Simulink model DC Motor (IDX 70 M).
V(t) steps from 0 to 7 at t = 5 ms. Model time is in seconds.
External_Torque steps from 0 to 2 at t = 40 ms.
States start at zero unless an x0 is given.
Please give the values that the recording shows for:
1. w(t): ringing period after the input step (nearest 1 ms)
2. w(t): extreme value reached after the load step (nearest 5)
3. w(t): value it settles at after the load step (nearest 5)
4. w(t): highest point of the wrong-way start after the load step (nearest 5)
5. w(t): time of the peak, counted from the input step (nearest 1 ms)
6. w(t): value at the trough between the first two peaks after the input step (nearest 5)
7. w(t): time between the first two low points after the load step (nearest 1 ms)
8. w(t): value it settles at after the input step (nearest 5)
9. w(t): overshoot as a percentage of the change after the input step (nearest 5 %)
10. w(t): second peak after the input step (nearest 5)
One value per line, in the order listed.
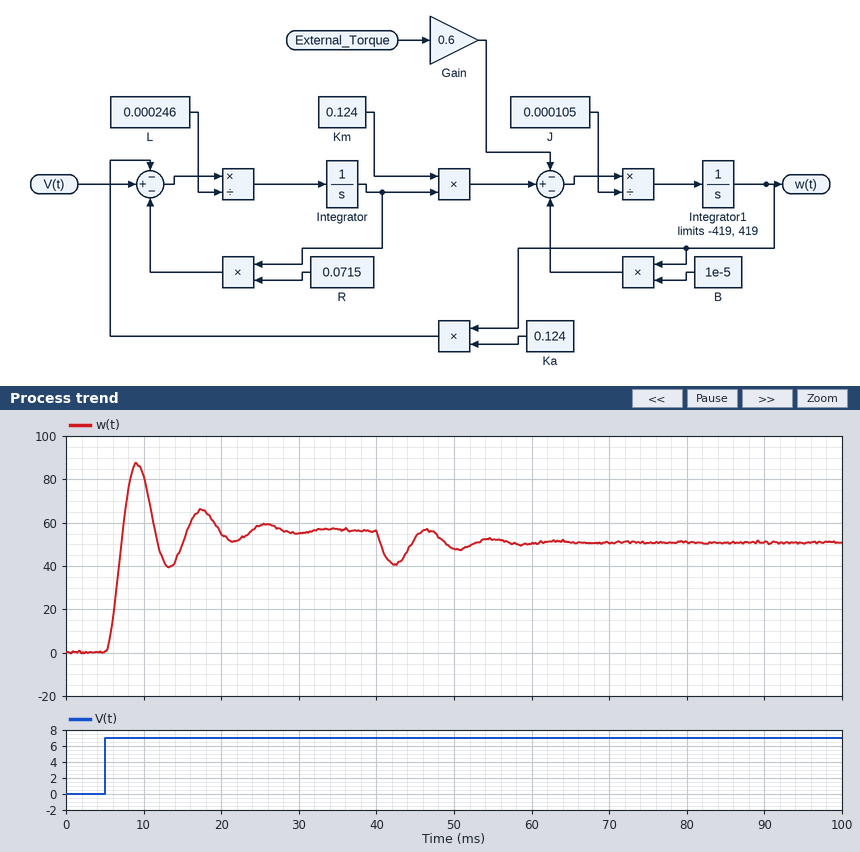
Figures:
8 ms
40
50
55
4 ms
40
8 ms
55
55 %
65
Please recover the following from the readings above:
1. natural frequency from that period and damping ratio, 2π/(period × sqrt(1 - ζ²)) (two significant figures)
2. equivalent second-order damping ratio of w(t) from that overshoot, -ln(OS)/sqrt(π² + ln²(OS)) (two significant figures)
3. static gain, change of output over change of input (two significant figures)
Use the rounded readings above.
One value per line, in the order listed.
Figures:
0.80 rad/ms
0.19
7.9
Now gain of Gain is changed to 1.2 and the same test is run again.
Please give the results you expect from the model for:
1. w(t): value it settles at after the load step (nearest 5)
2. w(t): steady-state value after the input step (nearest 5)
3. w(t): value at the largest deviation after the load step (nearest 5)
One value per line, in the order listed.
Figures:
45
55
25
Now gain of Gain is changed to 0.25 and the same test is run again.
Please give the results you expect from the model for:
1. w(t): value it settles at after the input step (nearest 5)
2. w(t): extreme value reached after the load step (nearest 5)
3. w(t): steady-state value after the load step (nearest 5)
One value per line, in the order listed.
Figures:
55
50
55
